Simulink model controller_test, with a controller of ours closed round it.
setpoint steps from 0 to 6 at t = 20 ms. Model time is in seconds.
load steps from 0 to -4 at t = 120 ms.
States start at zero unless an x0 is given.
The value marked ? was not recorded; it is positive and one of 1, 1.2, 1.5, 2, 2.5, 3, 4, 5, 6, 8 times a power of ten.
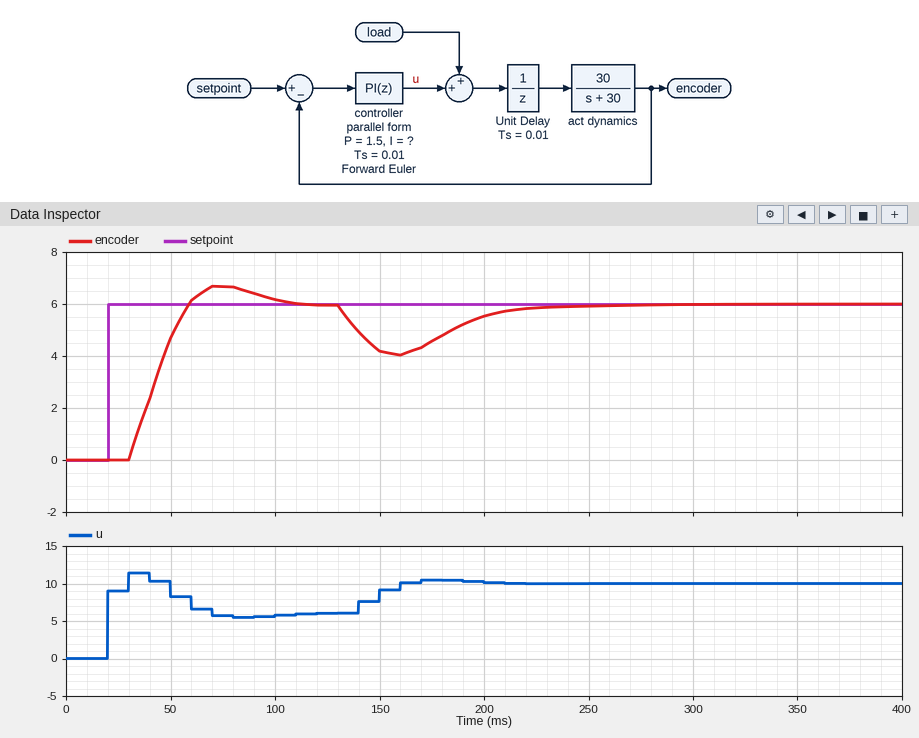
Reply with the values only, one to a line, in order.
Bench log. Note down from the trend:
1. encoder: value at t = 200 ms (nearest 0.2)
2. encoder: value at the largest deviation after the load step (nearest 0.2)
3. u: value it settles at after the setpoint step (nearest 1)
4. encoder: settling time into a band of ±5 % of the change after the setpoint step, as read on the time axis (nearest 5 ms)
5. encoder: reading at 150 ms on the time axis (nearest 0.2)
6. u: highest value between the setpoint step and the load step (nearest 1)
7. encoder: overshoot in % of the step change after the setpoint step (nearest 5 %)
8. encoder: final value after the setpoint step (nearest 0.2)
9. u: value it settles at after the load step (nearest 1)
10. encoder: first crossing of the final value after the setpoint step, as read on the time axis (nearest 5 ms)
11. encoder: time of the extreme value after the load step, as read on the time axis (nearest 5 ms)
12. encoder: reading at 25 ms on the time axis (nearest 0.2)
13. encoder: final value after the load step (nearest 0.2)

5.6
4.0
6
95 ms
4.2
11
10 %
6.0
10
60 ms
160 ms
0.0
6.0
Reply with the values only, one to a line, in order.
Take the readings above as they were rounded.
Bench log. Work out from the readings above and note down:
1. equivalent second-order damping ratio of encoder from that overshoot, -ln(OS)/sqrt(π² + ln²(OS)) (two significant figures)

0.59
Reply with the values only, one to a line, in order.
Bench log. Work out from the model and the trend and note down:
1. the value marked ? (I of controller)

40
